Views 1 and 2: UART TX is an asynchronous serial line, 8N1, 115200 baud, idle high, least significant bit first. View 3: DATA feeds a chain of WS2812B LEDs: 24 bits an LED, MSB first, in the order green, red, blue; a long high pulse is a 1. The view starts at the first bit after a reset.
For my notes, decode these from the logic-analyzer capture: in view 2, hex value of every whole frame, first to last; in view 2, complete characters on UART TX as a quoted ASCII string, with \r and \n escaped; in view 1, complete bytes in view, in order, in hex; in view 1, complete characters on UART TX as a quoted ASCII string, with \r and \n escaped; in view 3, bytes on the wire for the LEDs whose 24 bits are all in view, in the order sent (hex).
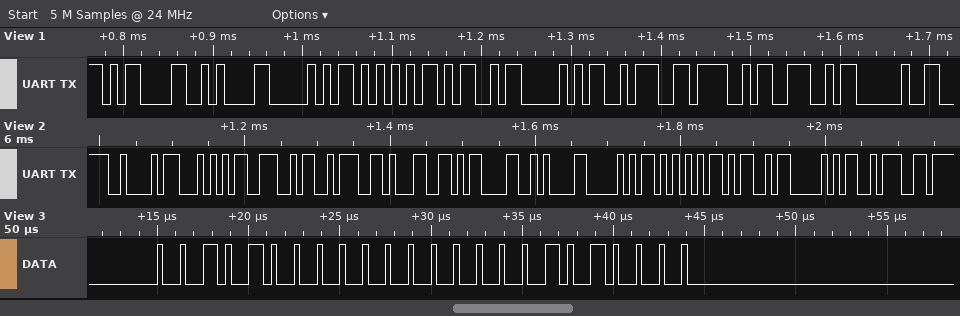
0x42 0x54 0x4E 0x3A 0x31 0x0D 0x0A 0x50 0x55 0x4D 0x50 0x3A
"BTN:1\r\nPUMP:"
0D 0A 50 55 4D 50 3A 4F 4E 20
"\r\nPUMP:ON "
28 00 50
